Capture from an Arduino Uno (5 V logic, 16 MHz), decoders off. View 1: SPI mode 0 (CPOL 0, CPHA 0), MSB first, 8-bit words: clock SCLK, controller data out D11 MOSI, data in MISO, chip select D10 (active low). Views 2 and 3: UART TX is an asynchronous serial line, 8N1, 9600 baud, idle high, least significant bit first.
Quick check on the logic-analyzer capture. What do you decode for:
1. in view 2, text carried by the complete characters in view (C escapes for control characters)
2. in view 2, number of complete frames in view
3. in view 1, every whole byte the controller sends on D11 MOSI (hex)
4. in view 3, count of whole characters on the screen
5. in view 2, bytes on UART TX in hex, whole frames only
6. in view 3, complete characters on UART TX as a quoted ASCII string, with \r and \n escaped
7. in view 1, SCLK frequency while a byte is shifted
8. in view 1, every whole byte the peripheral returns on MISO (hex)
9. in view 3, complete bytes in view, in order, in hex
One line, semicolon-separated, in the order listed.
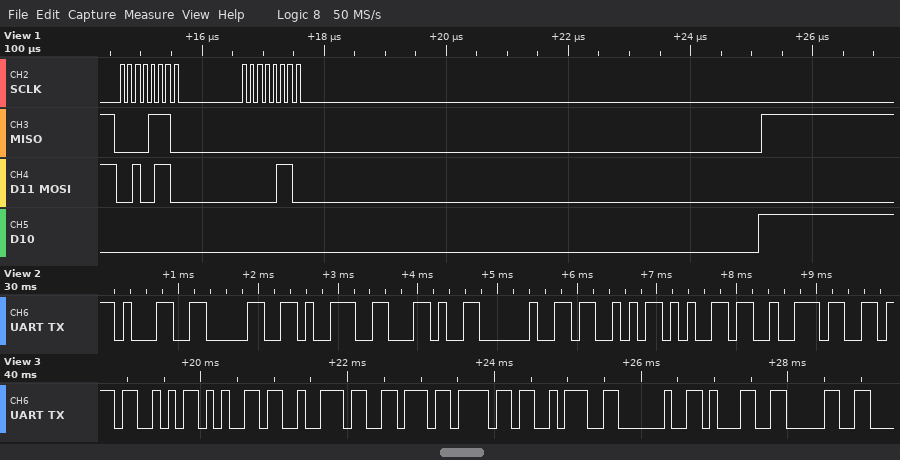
"109, Ser"; 8; 0x26 0x06; 9; 31 30 39 2C 20 53 65 72; "Servo: 10"; 8 MHz; 0x0E 0x00; 0x53 0x65 0x72 0x76 0x6F 0x3A 0x20 0x31 0x30
